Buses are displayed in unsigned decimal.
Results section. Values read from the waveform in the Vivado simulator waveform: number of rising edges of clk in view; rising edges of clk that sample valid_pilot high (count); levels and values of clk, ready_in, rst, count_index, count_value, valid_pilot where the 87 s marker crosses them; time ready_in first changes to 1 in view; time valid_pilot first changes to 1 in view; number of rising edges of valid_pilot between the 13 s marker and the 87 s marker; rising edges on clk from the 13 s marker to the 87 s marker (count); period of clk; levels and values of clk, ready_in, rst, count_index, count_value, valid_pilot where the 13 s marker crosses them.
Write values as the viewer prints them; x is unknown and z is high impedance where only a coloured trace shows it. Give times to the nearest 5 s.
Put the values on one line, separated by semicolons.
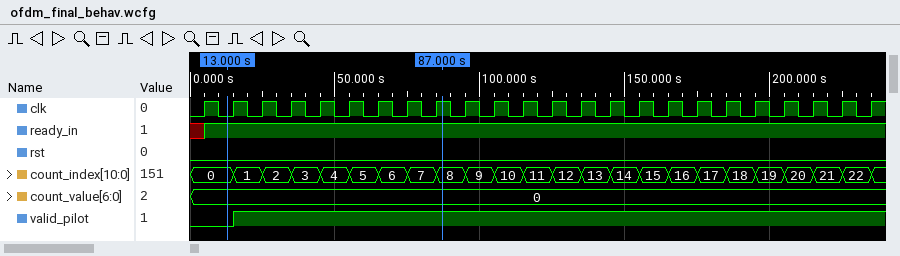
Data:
24; 22; clk=1, ready_in=1, rst=0, count_index=8, count_value=0, valid_pilot=1; 5 s; 15 s; 1; 8; 10 s; clk=0, ready_in=1, rst=0, count_index=0, count_value=0, valid_pilot=0
